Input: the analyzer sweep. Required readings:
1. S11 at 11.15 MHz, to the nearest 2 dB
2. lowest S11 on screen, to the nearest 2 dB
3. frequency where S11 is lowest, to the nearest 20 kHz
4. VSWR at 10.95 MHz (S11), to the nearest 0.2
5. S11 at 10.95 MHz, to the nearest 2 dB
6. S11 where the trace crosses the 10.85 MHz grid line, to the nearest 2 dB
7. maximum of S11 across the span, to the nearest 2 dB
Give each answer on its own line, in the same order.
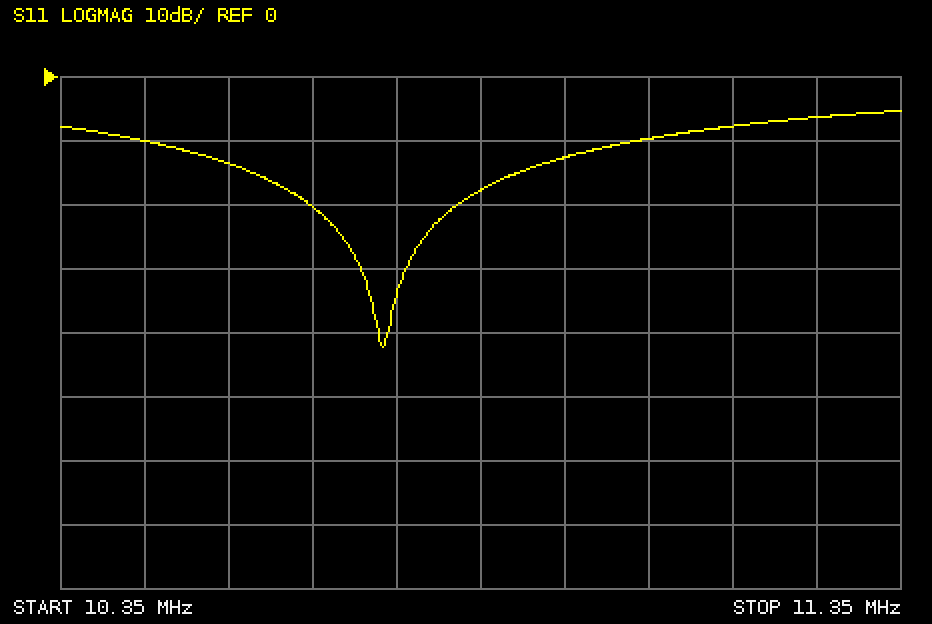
-8 dB
-42 dB
10.74 MHz
1.6
-12 dB
-18 dB
-6 dB
